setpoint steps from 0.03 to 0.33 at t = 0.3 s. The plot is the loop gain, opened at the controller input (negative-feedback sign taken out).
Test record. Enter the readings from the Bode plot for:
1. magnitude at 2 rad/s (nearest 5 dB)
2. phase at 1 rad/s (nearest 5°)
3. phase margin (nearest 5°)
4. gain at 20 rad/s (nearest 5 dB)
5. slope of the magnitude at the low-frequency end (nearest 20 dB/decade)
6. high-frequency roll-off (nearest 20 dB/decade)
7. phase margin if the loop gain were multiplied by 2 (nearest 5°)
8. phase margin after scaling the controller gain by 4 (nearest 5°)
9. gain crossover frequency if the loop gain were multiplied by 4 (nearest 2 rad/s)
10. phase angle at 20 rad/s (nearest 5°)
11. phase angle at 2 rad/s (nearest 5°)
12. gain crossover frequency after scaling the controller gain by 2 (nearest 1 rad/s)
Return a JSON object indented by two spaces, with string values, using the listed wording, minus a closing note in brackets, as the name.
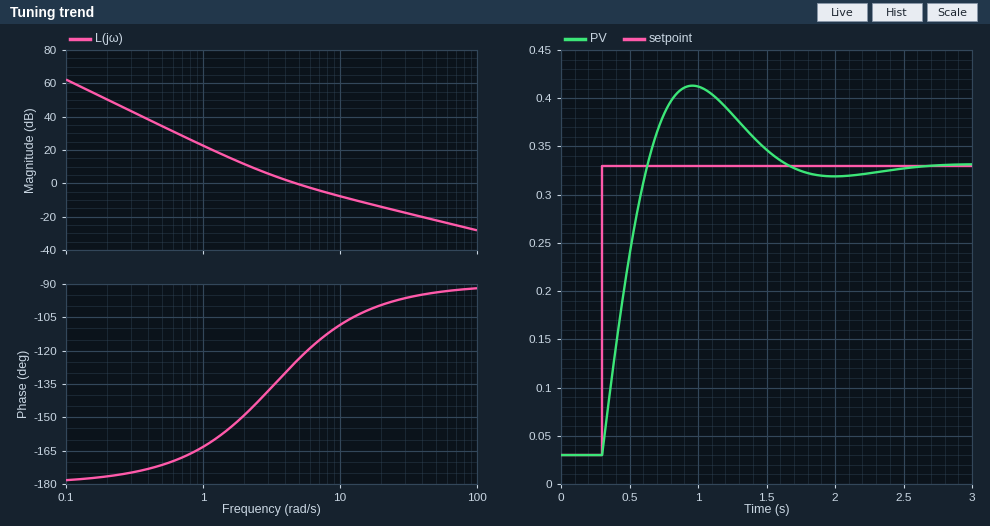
{
  "magnitude at 2 rad/s": "10 dB",
  "phase at 1 rad/s": "-165°",
  "phase margin": "55°",
  "gain at 20 rad/s": "-15 dB",
  "slope of the magnitude at the low-frequency end": "-40 dB/decade",
  "high-frequency roll-off": "-20 dB/decade",
  "phase margin if the loop gain were multiplied by 2": "70°",
  "phase margin after scaling the controller gain by 4": "80°",
  "gain crossover frequency if the loop gain were multiplied by 4": "16 rad/s",
  "phase angle at 20 rad/s": "-100°",
  "phase angle at 2 rad/s": "-150°",
  "gain crossover frequency after scaling the controller gain by 2": "8 rad/s"
}
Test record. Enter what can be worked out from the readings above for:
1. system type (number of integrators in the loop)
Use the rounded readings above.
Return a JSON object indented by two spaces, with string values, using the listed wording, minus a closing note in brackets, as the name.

{
  "system type": "2"
}
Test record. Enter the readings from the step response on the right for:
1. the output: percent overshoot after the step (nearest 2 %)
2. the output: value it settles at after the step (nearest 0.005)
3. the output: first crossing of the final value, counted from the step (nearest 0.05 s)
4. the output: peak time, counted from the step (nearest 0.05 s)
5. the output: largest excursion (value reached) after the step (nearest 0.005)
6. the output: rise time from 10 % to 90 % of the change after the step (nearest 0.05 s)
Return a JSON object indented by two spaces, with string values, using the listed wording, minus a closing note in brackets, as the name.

{
  "the output: percent overshoot after the step": "28 %",
  "the output: value it settles at after the step": "0.330",
  "the output: first crossing of the final value, counted from the step": "0.35 s",
  "the output: peak time, counted from the step": "0.65 s",
  "the output: largest excursion (value reached) after the step": "0.415",
  "the output: rise time from 10 % to 90 % of the change after the step": "0.25 s"
}
